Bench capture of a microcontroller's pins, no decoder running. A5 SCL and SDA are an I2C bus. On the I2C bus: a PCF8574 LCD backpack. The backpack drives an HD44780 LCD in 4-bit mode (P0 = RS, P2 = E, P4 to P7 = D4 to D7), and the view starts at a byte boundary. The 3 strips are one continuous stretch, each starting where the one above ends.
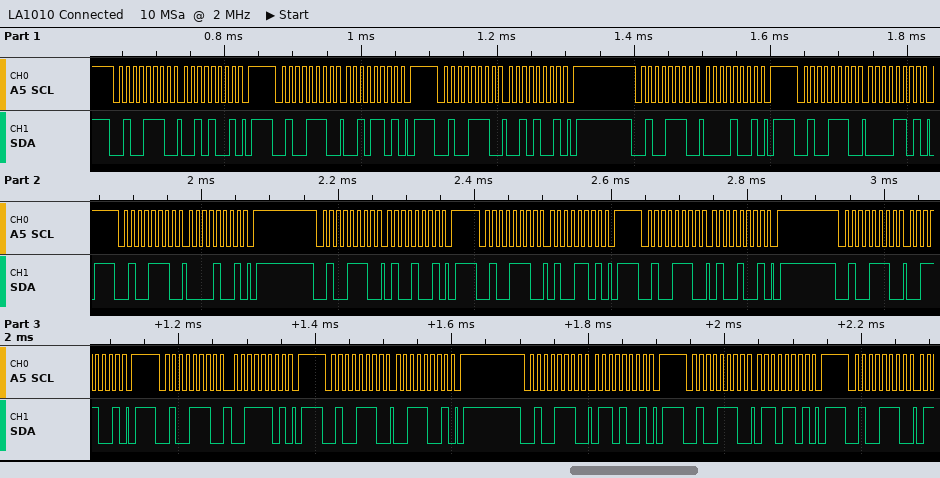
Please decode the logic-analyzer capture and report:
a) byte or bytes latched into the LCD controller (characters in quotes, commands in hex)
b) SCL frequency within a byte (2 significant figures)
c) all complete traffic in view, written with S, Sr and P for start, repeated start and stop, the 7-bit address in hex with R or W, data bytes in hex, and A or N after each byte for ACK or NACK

' ' 'C'
100 kHz
S 27W A 29 A P S 27W A 2D A P S 27W A 29 A P S 27W A 09 A P S 27W A 0D A P S 27W A 09 A P S 27W A 49 A P S 27W A 4D A P S 27W A 49 A P S 27W A 39 A P S 27W A 3D A P S 27W A 39 A P S 27W A 69 A P S 27W A 6D A P S 27W A
